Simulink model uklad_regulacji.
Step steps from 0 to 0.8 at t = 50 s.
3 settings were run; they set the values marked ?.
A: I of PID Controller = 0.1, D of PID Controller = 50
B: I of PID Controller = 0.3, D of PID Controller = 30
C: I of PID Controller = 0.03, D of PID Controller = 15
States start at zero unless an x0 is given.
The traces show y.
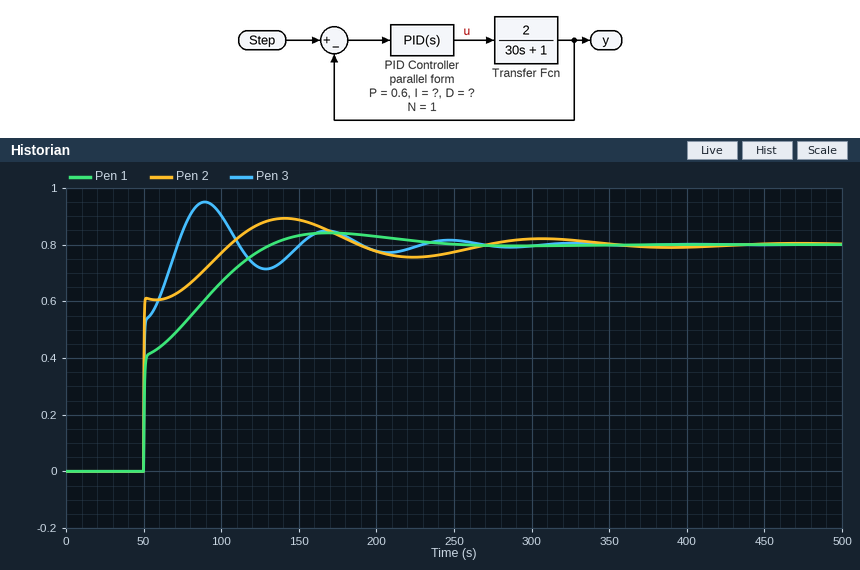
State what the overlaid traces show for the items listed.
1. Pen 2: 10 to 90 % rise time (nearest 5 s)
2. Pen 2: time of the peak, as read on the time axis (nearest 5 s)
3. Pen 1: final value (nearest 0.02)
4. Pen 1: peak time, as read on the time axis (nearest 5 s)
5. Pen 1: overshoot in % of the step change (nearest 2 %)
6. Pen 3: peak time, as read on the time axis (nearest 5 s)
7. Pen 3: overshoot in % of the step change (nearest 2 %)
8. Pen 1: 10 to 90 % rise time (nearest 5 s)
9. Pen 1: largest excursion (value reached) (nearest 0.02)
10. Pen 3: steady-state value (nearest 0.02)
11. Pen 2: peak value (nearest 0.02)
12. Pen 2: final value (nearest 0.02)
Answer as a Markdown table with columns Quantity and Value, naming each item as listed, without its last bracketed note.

| Quantity | Value |
|---|---|
| Pen 2: 10 to 90 % rise time | 40 s |
| Pen 2: time of the peak, as read on the time axis | 140 s |
| Pen 1: final value | 0.80 |
| Pen 1: peak time, as read on the time axis | 170 s |
| Pen 1: overshoot in % of the step change | 6 % |
| Pen 3: peak time, as read on the time axis | 90 s |
| Pen 3: overshoot in % of the step change | 18 % |
| Pen 1: 10 to 90 % rise time | 60 s |
| Pen 1: largest excursion (value reached) | 0.84 |
| Pen 3: steady-state value | 0.80 |
| Pen 2: peak value | 0.90 |
| Pen 2: final value | 0.80 |
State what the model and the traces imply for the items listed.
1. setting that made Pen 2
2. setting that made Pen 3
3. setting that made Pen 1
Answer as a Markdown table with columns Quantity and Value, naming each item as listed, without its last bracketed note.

| Quantity | Value |
|---|---|
| setting that made Pen 2 | A |
| setting that made Pen 3 | B |
| setting that made Pen 1 | C |
